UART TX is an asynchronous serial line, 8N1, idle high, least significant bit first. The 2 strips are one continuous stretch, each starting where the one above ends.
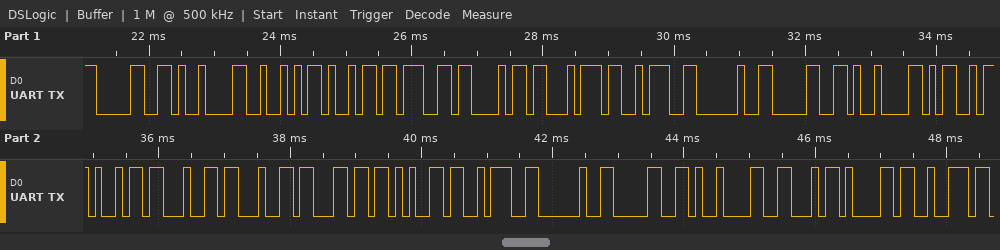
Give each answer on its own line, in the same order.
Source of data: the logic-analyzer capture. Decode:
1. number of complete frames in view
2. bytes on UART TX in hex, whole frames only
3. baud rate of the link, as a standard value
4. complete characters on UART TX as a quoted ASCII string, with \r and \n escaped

24
30 09 52 69 67 68 74 3A 20 30 09 4D 69 64 64 6C 65 3A 20 30 09 46 61 72
9600 baud
"0\tRight: 0\tMiddle: 0\tFar"
